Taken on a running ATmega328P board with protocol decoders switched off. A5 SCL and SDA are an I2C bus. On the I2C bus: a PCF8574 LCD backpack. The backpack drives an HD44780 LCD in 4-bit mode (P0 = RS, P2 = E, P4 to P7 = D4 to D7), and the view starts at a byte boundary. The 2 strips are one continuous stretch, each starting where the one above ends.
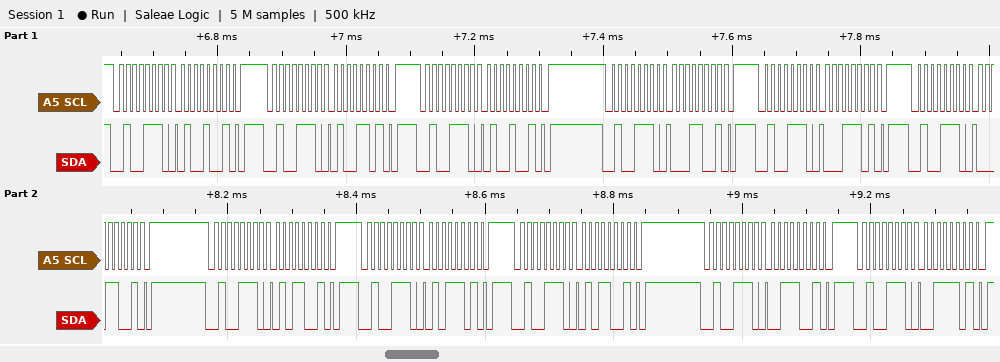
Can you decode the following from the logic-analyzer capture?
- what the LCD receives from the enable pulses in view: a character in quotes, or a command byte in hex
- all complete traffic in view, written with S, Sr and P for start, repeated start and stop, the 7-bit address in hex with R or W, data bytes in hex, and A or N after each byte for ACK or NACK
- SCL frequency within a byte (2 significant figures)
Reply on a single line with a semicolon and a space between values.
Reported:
'A'; S 27W A 49 A P S 27W A 4D A P S 27W A 49 A P S 27W A 19 A P S 27W A 1D A P S 27W A 19 A P S 27W A 59 A P S 27W A 5D A P S 27W A 59 A P S 27W A 39 A P S 27W A 3D A P; 100 kHz
